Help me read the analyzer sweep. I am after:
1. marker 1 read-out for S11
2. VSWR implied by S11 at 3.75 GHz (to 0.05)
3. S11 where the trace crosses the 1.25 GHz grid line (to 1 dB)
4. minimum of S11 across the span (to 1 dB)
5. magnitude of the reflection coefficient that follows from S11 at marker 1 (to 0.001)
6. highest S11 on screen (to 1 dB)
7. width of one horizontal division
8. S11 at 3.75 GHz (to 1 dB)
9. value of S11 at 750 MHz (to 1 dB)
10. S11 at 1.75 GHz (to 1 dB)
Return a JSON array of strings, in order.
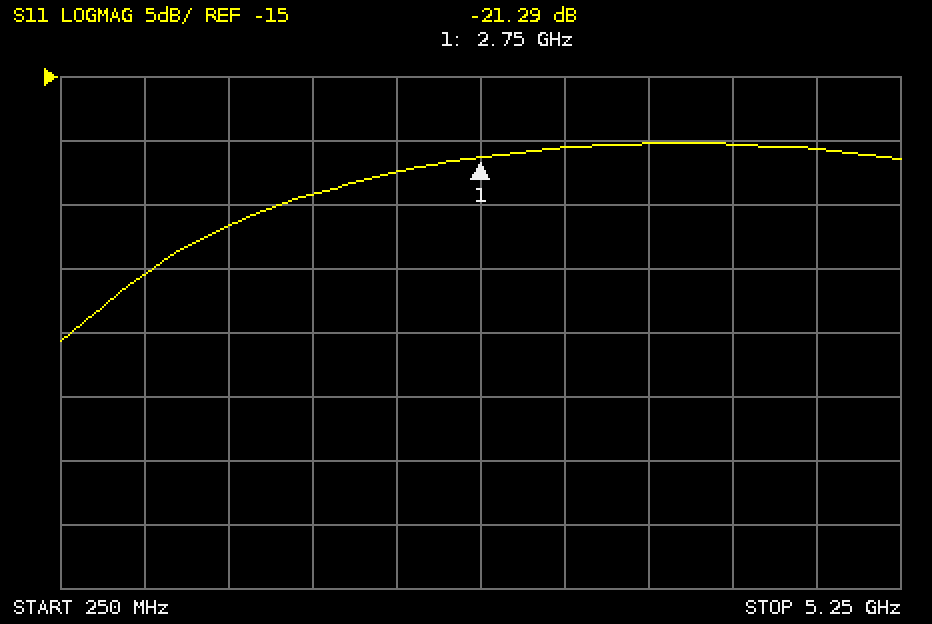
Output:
["-21.29 dB", "1.20", "-27 dB", "-36 dB", "0.086", "-20 dB", "500 MHz", "-20 dB", "-30 dB", "-24 dB"]
